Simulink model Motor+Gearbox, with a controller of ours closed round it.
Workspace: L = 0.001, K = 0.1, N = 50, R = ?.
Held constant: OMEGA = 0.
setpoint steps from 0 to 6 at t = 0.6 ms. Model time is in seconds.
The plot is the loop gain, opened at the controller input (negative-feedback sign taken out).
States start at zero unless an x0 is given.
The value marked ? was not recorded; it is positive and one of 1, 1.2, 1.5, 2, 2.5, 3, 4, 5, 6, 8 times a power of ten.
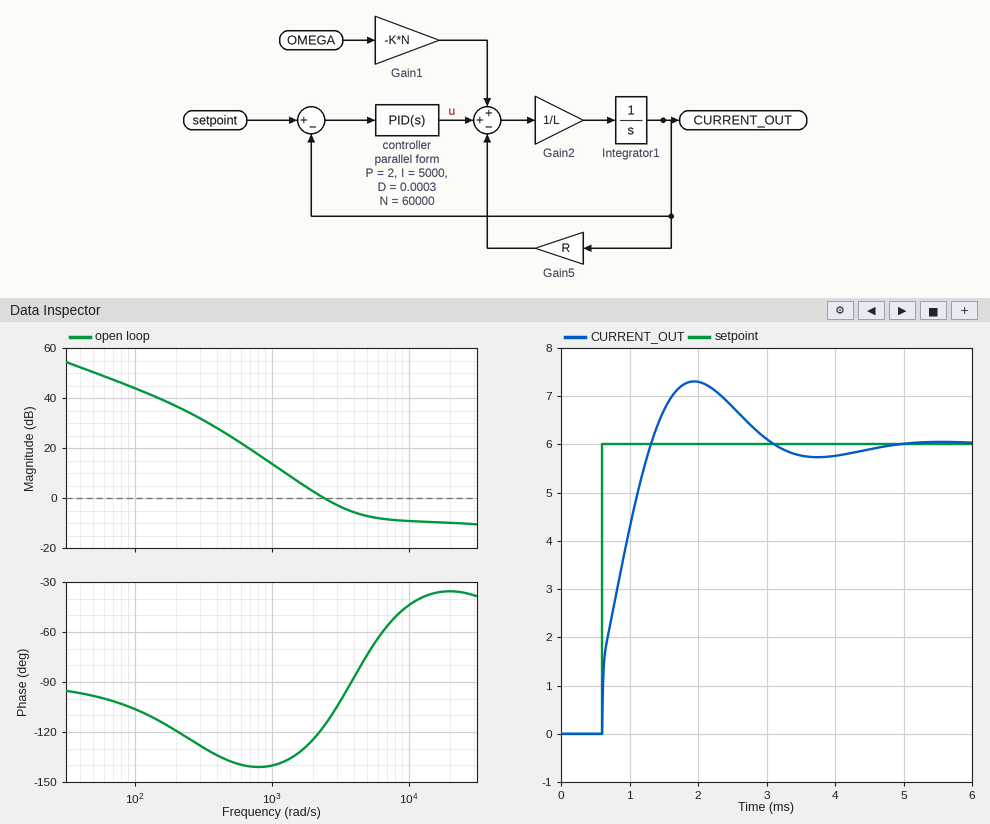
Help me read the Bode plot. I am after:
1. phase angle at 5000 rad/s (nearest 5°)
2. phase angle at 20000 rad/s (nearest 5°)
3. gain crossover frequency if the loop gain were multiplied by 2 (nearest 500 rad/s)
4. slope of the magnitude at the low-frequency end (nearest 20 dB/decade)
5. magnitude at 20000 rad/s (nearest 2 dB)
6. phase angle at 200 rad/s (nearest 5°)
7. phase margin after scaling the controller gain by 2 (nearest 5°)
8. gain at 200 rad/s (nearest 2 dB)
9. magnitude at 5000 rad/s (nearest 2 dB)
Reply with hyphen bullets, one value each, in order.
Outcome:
- -75°
- -35°
- 4000 rad/s
- -20 dB/decade
- -10 dB
- -120°
- 95°
- 36 dB
- -8 dB
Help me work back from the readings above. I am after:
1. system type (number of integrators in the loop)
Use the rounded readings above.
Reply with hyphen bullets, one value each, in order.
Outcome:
- 1
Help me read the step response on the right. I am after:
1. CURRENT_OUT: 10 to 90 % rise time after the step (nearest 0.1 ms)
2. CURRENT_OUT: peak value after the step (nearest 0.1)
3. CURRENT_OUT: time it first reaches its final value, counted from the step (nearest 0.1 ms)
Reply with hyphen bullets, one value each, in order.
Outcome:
- 0.6 ms
- 7.3
- 0.7 ms
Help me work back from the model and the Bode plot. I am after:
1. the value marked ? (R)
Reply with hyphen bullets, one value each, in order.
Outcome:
- 0.3
